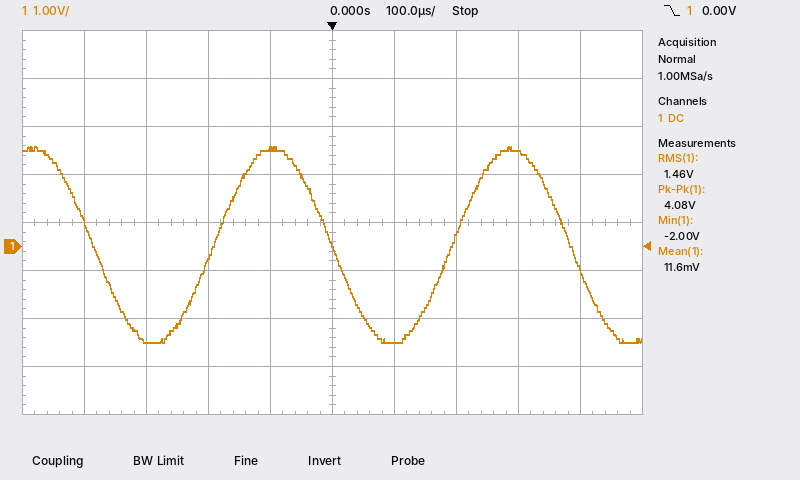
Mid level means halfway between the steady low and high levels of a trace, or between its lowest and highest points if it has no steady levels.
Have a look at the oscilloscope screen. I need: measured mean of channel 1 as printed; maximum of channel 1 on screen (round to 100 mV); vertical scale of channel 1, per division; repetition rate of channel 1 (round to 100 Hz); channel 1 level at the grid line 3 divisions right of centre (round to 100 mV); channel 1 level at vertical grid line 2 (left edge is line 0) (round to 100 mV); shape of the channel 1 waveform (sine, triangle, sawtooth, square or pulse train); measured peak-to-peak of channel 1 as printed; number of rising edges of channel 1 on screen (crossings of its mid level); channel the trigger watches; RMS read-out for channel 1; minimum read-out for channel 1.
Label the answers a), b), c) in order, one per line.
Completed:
a) 11.6 mV
b) 2.1 V
c) 1 V
d) 2.6 kHz
e) 2.0 V
f) -2.0 V
g) sine
h) 4.08 V
i) 2
j) channel 1
k) 1.46 V
l) -2.00 V
